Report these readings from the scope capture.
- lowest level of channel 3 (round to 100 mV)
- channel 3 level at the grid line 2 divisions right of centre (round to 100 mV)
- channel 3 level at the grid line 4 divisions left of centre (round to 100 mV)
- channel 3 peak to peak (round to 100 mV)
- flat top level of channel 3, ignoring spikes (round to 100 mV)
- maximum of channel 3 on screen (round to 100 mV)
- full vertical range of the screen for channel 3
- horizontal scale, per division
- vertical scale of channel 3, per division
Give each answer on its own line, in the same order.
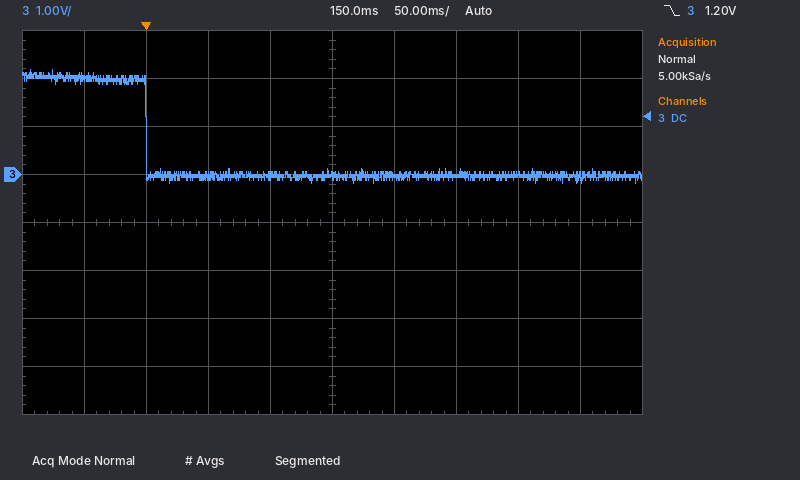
-200 mV
0.0 V
2.0 V
2.4 V
2.0 V
2.2 V
8 V
50 ms
1 V
